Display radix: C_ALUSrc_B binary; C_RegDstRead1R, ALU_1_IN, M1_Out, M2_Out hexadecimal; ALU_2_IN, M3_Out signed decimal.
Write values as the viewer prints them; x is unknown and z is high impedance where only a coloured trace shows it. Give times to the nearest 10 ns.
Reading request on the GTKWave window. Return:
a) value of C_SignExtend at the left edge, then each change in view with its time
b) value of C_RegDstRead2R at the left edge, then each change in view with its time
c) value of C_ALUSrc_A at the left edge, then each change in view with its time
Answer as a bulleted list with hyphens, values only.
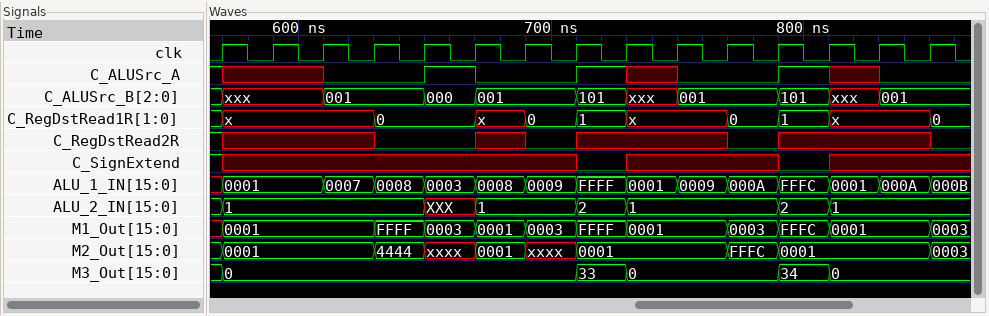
- 1, x at 570 ns, 0 at 710 ns, x at 730 ns, 0 at 790 ns, x at 810 ns
- 1, x at 570 ns, 0 at 630 ns, x at 670 ns, 0 at 690 ns, x at 710 ns, 0 at 770 ns, x at 790 ns, 0 at 850 ns
- 1, x at 570 ns, 0 at 610 ns, 1 at 650 ns, 0 at 670 ns, 1 at 710 ns, x at 730 ns, 0 at 750 ns, 1 at 790 ns, x at 810 ns, 0 at 830 ns
